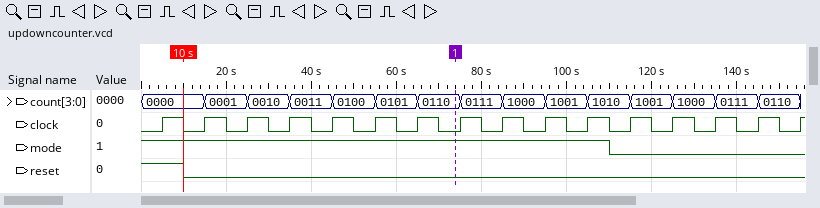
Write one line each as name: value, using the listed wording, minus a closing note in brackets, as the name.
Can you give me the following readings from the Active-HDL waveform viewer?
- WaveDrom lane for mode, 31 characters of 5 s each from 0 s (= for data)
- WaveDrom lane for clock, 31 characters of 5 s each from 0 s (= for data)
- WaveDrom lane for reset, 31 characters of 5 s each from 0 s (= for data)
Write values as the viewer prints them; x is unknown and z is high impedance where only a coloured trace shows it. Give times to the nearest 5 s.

WaveDrom lane for mode, 31 characters of 5 s each from 0 s: {name: 'mode', wave: '1.....................0........'}
WaveDrom lane for clock, 31 characters of 5 s each from 0 s: {name: 'clock', wave: '0101010101010101010101010101010'}
WaveDrom lane for reset, 31 characters of 5 s each from 0 s: {name: 'reset', wave: '1.0............................'}
